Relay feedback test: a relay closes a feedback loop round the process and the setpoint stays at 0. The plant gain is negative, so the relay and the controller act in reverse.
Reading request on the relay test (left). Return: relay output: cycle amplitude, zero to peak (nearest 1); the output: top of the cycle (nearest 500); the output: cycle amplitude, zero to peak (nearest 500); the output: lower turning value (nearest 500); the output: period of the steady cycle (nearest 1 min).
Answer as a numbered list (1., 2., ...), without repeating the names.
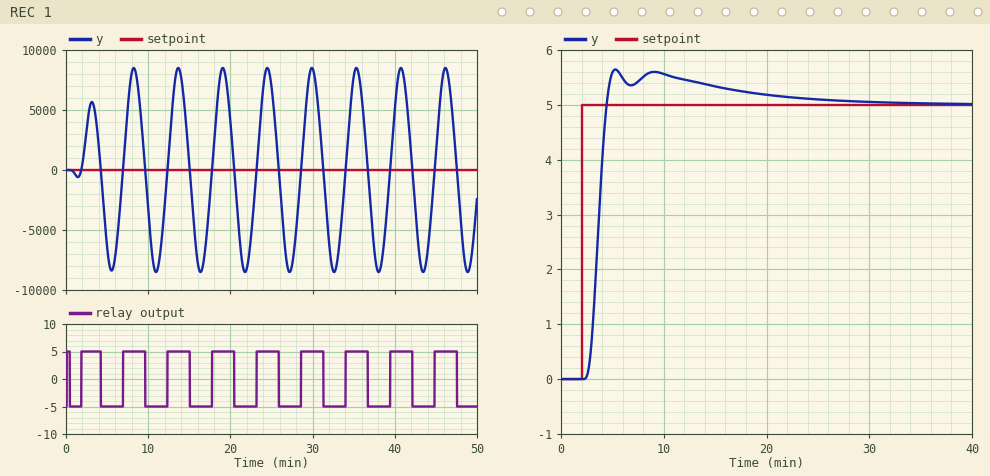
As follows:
1. 5
2. 8500
3. 8500
4. -8500
5. 5 min
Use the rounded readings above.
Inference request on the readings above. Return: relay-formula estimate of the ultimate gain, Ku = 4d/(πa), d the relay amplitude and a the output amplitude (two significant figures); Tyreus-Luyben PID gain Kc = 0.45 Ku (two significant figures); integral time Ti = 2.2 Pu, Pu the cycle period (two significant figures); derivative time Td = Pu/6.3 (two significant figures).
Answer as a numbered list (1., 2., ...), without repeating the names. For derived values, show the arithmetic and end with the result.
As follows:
1. 4 × 5 / (π × 8500) = 0.00075
2. 0.45 × 0.00075 = 0.00034
3. 2.2 × 5 = 11 min
4. 5 / 6.3 = 0.79 min
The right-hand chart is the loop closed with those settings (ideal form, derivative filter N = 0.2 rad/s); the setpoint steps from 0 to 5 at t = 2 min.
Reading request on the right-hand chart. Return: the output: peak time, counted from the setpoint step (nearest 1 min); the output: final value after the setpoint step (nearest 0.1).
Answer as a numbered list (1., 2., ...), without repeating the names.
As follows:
1. 3 min
2. 5.0
